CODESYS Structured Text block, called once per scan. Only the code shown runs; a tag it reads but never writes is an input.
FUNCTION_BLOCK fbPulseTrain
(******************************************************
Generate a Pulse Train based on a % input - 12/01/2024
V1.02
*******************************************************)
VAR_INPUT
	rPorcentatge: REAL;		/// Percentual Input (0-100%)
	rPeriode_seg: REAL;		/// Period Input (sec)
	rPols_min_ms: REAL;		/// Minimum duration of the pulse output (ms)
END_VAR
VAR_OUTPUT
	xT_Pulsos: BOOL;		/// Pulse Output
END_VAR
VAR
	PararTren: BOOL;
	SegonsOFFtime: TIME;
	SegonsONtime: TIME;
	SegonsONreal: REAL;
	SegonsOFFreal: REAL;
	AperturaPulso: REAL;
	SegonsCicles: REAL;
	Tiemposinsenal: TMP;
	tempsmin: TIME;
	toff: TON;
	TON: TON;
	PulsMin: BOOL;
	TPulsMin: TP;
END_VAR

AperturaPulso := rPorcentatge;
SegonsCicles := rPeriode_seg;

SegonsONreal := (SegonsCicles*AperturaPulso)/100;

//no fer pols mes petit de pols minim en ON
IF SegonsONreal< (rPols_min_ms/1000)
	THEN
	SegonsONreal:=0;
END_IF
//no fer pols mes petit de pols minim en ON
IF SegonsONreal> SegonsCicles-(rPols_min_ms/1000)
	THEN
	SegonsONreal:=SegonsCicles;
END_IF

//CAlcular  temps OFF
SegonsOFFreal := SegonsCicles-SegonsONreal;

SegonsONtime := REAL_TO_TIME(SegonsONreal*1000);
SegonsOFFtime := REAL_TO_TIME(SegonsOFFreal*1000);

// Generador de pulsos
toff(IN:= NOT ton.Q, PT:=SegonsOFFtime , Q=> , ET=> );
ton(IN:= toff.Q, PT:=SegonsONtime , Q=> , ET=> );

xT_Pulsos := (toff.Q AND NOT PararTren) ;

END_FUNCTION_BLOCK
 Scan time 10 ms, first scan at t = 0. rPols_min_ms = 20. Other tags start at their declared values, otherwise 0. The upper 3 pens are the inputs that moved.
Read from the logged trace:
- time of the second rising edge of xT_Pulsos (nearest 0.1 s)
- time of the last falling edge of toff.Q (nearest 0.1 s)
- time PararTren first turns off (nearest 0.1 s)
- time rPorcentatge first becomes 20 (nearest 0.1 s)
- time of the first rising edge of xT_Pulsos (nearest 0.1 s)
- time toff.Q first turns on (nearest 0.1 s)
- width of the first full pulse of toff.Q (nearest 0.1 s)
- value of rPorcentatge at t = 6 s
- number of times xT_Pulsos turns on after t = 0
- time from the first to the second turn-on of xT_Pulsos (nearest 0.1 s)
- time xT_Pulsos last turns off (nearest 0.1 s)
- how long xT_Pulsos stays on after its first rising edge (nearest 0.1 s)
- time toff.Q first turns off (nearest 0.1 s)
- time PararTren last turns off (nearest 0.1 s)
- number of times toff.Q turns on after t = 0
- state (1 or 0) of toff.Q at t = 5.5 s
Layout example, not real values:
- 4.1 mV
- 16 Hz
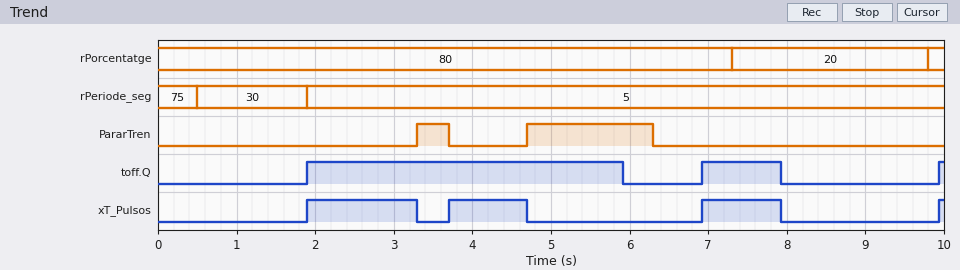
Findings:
- 3.7 s
- 7.9 s
- 3.7 s
- 7.3 s
- 1.9 s
- 1.9 s
- 4.0 s
- 80
- 4
- 1.8 s
- 7.9 s
- 1.4 s
- 5.9 s
- 6.3 s
- 3
- 1
